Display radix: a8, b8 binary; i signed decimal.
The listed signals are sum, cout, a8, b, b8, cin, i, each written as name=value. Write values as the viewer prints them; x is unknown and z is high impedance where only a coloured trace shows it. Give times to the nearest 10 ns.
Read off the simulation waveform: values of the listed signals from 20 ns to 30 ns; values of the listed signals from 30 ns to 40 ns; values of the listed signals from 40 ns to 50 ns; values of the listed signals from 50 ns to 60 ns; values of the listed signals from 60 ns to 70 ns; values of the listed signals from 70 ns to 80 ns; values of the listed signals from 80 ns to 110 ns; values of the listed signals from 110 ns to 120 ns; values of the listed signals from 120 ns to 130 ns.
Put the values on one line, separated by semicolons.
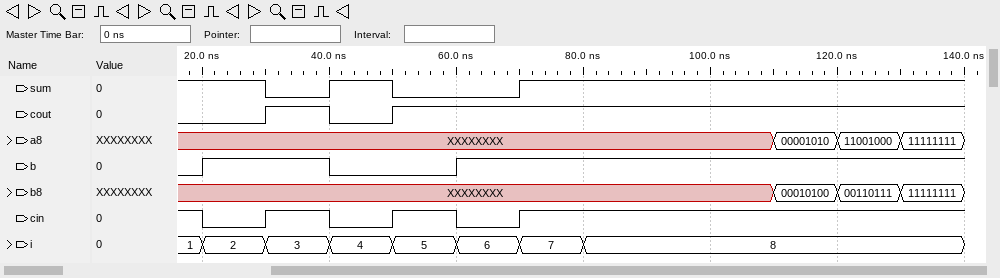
sum=1, cout=0, a8=XXXXXXXX, b=1, b8=XXXXXXXX, cin=0, i=2; sum=0, cout=1, a8=XXXXXXXX, b=1, b8=XXXXXXXX, cin=1, i=3; sum=1, cout=0, a8=XXXXXXXX, b=0, b8=XXXXXXXX, cin=0, i=4; sum=0, cout=1, a8=XXXXXXXX, b=0, b8=XXXXXXXX, cin=1, i=5; sum=0, cout=1, a8=XXXXXXXX, b=1, b8=XXXXXXXX, cin=0, i=6; sum=1, cout=1, a8=XXXXXXXX, b=1, b8=XXXXXXXX, cin=1, i=7; sum=1, cout=1, a8=XXXXXXXX, b=1, b8=XXXXXXXX, cin=1, i=8; sum=1, cout=1, a8=00001010, b=1, b8=00010100, cin=1, i=8; sum=1, cout=1, a8=11001000, b=1, b8=00110111, cin=1, i=8
